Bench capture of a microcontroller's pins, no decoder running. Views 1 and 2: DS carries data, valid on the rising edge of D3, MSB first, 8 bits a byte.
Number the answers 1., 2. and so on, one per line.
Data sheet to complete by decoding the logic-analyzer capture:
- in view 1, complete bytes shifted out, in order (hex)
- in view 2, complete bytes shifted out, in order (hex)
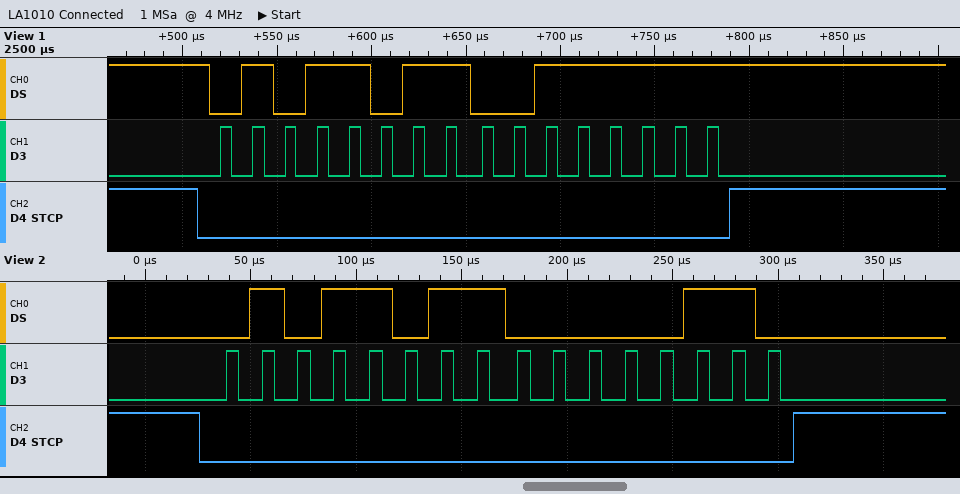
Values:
1. 5B 3F
2. 5B 06
